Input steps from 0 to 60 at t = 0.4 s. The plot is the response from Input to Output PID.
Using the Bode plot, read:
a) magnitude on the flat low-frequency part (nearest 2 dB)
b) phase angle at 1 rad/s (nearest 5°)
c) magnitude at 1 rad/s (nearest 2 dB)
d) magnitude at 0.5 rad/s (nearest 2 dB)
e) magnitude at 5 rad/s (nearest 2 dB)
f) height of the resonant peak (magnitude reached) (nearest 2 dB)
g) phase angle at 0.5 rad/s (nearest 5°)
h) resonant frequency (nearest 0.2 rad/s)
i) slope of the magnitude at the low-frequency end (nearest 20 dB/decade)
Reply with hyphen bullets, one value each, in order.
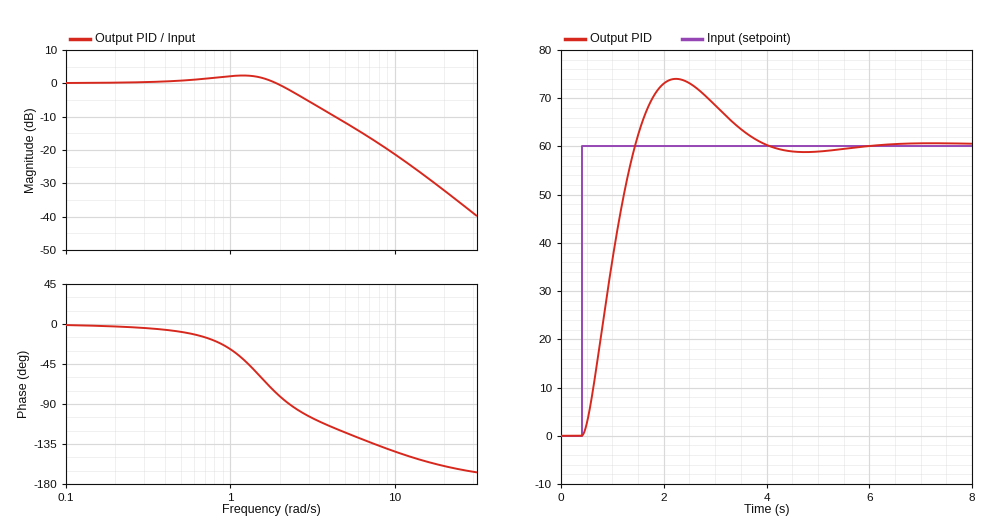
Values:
- 0 dB
- -30°
- 2 dB
- 0 dB
- -12 dB
- 2 dB
- -10°
- 1.2 rad/s
- 0 dB/decade
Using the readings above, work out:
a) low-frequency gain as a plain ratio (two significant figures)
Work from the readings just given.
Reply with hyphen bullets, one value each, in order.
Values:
- 1.0
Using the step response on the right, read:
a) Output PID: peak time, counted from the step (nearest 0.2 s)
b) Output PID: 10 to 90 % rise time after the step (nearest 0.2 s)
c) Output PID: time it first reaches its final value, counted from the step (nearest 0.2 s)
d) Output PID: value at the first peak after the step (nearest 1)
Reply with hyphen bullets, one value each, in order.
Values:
- 1.8 s
- 0.8 s
- 1.0 s
- 74
